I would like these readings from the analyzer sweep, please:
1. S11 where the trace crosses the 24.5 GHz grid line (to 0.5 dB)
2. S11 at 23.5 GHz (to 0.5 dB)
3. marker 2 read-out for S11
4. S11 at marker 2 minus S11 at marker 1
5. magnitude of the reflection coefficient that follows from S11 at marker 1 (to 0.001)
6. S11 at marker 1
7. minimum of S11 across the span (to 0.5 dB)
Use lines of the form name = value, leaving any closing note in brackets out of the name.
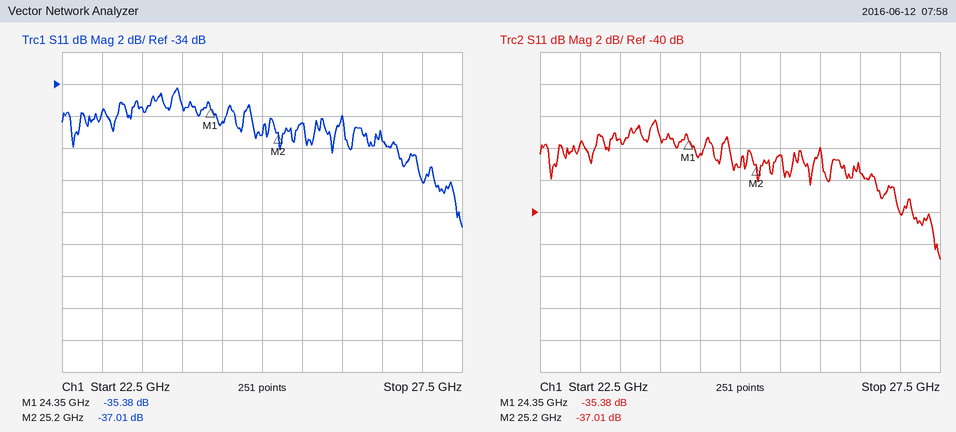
S11 where the trace crosses the 24.5 GHz grid line = -36.5 dB
S11 at 23.5 GHz = -35.5 dB
marker 2 read-out for S11 = -37.01 dB
S11 at marker 2 minus S11 at marker 1 = -1.63 dB
magnitude of the reflection coefficient that follows from S11 at marker 1 = 0.017
S11 at marker 1 = -35.38 dB
minimum of S11 across the span = -43.0 dB
